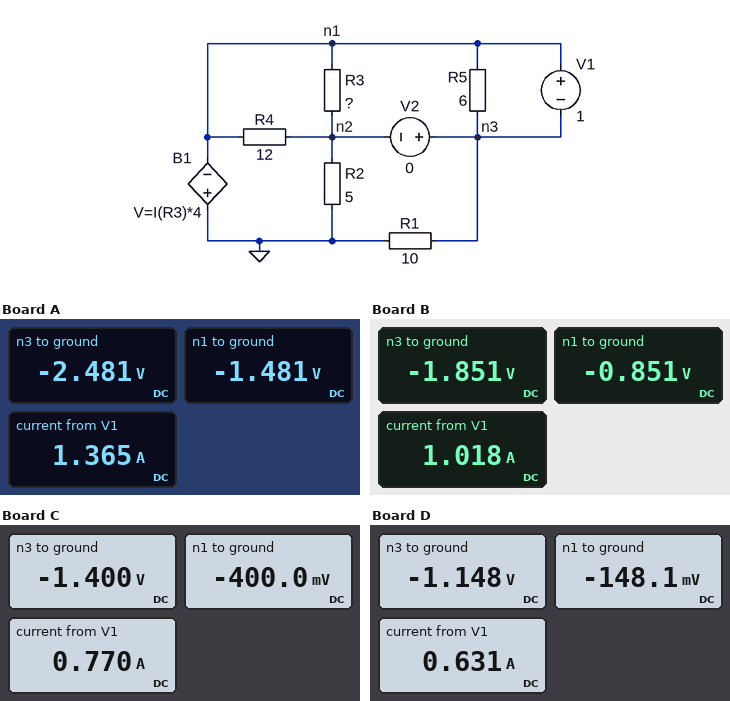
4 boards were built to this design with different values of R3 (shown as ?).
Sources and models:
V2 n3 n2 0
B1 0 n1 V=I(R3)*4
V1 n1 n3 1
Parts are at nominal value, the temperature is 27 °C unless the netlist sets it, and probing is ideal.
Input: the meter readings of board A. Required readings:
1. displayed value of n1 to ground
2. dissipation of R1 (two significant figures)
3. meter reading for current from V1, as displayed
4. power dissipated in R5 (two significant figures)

-1.481 V
620 mW
1.365 A
170 mW
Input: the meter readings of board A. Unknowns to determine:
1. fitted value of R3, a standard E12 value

2.7 Ω
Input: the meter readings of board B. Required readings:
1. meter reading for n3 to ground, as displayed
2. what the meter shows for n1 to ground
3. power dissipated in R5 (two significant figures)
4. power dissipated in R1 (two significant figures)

-1.851 V
-0.851 V
170 mW
340 mW
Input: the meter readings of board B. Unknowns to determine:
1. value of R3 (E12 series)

4.7 Ω
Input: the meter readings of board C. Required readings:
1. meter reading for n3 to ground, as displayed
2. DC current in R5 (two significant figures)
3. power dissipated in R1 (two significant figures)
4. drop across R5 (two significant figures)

-1.400 V
170 mA
200 mW
1.0 V
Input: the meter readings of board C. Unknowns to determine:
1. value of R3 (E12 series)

10 Ω
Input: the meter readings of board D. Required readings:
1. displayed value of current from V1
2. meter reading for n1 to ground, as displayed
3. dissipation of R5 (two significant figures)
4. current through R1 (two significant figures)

0.631 A
-148.1 mV
170 mW
110 mA
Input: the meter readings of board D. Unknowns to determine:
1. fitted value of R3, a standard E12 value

27 Ω
